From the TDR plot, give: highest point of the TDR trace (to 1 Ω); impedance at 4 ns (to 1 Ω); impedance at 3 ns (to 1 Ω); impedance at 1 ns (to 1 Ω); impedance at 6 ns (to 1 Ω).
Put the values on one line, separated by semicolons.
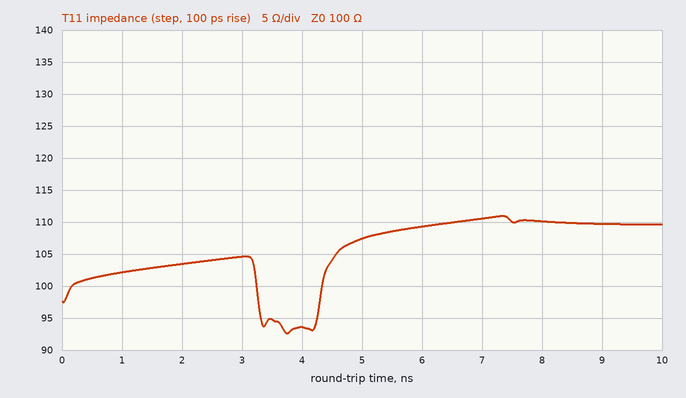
111 Ω; 94 Ω; 105 Ω; 102 Ω; 109 Ω
